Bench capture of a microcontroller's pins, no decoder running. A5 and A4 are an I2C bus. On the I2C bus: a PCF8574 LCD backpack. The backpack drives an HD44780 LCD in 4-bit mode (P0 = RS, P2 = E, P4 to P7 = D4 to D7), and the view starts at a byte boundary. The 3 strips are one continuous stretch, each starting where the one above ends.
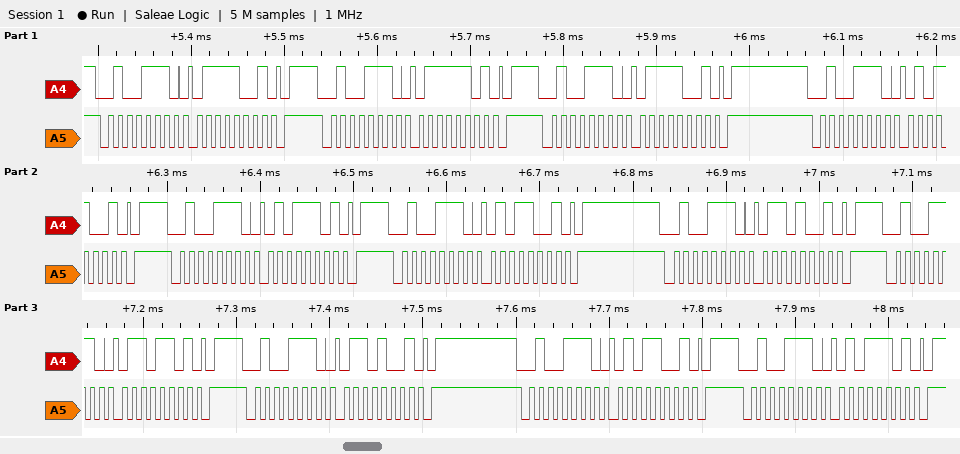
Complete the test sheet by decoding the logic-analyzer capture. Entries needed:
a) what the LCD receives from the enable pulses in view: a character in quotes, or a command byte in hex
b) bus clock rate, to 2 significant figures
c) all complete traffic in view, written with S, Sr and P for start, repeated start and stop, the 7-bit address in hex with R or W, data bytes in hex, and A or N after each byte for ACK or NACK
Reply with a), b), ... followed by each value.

a) 'u'
b) 100 kHz
c) S 27W A 79 A P S 27W A 7D A P S 27W A 79 A P S 27W A 59 A P S 27W A 5D A P S 27W A 59 A P S 27W A 69 A P S 27W A 6D A P S 27W A 69 A P S 27W A 59 A P S 27W A 5D A P
